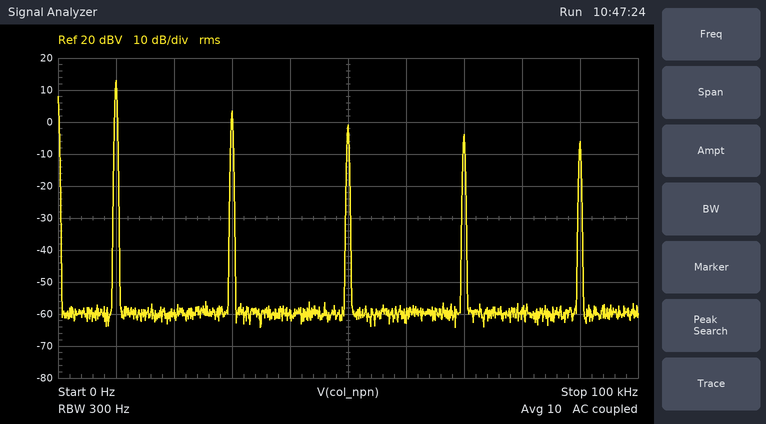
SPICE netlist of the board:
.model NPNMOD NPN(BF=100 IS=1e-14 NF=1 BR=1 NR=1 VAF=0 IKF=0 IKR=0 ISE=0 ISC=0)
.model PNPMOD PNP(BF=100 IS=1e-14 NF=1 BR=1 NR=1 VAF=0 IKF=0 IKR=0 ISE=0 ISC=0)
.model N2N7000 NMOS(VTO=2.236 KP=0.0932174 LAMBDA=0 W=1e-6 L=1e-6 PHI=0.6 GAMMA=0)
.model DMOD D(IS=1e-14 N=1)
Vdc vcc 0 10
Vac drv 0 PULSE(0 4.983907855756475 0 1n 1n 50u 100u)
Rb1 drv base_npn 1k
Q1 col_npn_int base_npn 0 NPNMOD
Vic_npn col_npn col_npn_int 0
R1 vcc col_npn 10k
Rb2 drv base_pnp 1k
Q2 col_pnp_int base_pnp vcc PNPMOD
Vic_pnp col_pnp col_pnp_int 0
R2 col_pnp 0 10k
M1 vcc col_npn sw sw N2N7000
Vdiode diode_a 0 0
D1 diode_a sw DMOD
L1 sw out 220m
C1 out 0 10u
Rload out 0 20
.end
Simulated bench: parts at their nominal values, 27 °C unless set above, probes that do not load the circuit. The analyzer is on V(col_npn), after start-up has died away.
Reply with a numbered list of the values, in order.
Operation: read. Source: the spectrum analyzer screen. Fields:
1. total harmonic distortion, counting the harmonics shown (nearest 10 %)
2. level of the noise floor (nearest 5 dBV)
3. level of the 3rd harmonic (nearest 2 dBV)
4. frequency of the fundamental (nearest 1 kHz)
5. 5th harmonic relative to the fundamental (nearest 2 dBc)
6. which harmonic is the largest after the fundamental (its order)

1. 40 %
2. -60 dBV
3. 4 dBV
4. 10 kHz
5. -14 dBc
6. 3
